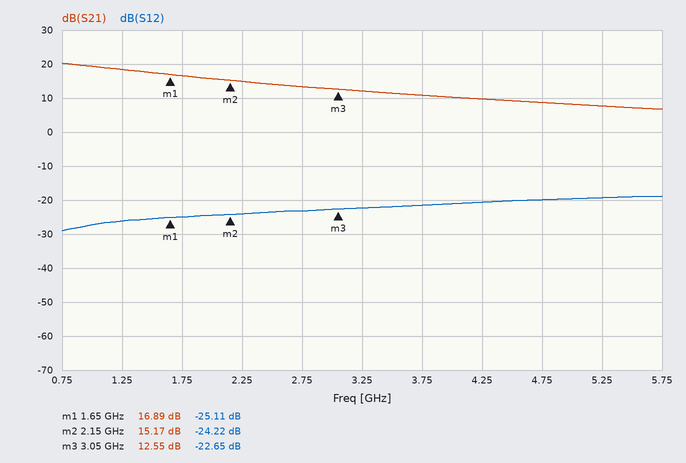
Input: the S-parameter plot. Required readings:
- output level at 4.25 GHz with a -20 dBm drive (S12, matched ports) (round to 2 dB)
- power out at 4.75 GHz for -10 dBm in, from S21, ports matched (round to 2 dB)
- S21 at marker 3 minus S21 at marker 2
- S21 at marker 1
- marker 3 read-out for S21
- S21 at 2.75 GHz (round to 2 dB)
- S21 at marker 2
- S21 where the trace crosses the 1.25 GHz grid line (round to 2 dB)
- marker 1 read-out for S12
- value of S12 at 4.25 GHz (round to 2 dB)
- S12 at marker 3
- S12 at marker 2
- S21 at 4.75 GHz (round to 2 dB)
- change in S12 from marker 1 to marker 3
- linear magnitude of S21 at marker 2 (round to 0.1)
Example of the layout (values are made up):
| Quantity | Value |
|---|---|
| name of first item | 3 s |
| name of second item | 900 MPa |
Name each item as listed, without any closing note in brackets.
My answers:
| Quantity | Value |
|---|---|
| output level at 4.25 GHz with a -20 dBm drive (S12, matched ports) | -40 dBm |
| power out at 4.75 GHz for -10 dBm in, from S21, ports matched | -2 dBm |
| S21 at marker 3 minus S21 at marker 2 | -2.62 dB |
| S21 at marker 1 | 16.89 dB |
| marker 3 read-out for S21 | 12.55 dB |
| S21 at 2.75 GHz | 14 dB |
| S21 at marker 2 | 15.17 dB |
| S21 where the trace crosses the 1.25 GHz grid line | 18 dB |
| marker 1 read-out for S12 | -25.11 dB |
| value of S12 at 4.25 GHz | -20 dB |
| S12 at marker 3 | -22.65 dB |
| S12 at marker 2 | -24.22 dB |
| S21 at 4.75 GHz | 8 dB |
| change in S12 from marker 1 to marker 3 | 2.46 dB |
| linear magnitude of S21 at marker 2 | 5.7 |
